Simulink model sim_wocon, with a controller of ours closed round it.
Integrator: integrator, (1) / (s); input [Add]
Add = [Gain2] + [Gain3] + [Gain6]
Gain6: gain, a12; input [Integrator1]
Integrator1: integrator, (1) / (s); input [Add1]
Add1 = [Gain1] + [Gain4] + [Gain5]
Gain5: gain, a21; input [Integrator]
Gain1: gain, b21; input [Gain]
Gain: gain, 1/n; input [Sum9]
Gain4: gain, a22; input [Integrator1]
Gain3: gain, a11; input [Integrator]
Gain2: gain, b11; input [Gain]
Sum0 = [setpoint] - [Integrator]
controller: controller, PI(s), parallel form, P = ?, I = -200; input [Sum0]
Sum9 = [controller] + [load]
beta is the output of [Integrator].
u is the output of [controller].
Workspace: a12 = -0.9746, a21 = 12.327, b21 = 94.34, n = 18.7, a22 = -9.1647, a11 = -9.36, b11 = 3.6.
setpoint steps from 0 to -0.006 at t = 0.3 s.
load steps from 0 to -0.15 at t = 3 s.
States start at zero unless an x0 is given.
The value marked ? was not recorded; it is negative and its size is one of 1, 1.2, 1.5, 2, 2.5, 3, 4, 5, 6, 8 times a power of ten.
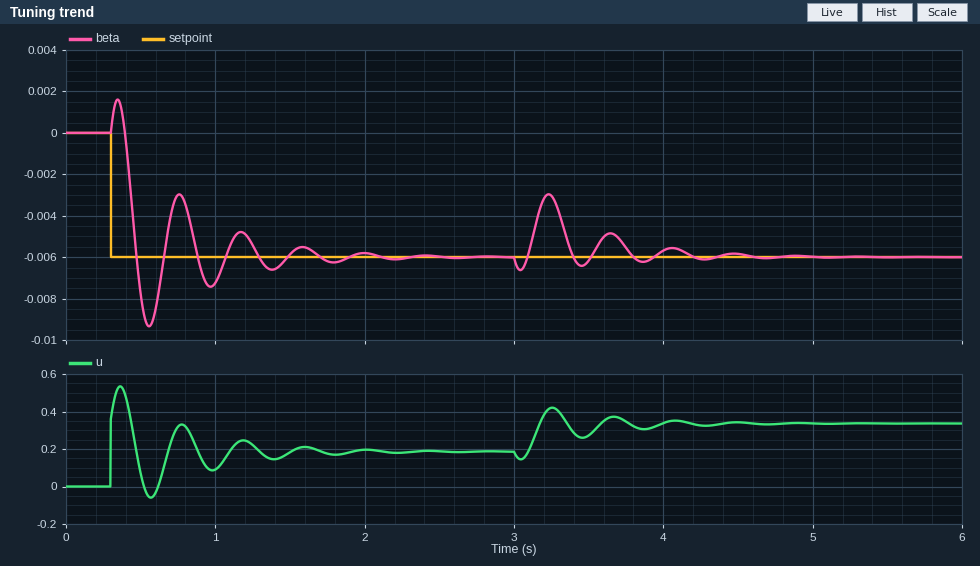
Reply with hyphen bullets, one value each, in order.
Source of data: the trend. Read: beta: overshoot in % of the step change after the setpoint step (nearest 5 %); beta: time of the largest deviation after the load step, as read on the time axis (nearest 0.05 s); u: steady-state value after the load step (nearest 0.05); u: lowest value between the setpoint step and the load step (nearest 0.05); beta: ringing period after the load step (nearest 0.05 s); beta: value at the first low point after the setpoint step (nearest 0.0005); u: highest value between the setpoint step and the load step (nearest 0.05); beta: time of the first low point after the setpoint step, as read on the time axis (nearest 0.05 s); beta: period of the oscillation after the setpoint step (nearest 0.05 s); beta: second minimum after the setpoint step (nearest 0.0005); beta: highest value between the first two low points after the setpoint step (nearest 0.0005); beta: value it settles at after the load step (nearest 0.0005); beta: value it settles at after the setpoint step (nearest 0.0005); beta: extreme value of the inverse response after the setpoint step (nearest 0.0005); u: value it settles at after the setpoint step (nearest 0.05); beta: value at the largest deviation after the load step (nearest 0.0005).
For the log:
- 55 %
- 3.25 s
- 0.35
- -0.05
- 0.40 s
- -0.0095
- 0.55
- 0.55 s
- 0.40 s
- -0.0075
- -0.0030
- -0.0060
- -0.0060
- 0.0015
- 0.20
- -0.0030
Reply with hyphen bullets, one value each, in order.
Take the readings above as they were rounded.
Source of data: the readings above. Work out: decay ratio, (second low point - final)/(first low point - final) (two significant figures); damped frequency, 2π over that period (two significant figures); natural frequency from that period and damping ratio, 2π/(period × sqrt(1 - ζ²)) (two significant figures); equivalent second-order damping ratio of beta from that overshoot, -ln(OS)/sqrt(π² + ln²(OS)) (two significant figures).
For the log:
- 0.43
- 16 rad/s
- 16 rad/s
- 0.19
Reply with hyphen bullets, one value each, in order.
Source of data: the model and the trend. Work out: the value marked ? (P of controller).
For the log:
- -60
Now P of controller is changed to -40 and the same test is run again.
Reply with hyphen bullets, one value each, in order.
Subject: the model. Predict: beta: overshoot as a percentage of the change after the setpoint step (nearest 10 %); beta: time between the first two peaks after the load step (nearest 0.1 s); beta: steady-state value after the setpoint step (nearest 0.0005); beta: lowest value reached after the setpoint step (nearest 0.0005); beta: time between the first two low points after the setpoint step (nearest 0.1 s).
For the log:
- 30 %
- 0.5 s
- -0.0060
- -0.0080
- 0.5 s
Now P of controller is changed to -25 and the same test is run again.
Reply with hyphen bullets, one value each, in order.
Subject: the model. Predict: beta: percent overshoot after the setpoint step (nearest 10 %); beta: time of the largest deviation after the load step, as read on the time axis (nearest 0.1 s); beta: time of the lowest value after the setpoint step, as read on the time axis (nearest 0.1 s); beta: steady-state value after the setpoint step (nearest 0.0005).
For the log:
- 30 %
- 3.3 s
- 0.7 s
- -0.0060
